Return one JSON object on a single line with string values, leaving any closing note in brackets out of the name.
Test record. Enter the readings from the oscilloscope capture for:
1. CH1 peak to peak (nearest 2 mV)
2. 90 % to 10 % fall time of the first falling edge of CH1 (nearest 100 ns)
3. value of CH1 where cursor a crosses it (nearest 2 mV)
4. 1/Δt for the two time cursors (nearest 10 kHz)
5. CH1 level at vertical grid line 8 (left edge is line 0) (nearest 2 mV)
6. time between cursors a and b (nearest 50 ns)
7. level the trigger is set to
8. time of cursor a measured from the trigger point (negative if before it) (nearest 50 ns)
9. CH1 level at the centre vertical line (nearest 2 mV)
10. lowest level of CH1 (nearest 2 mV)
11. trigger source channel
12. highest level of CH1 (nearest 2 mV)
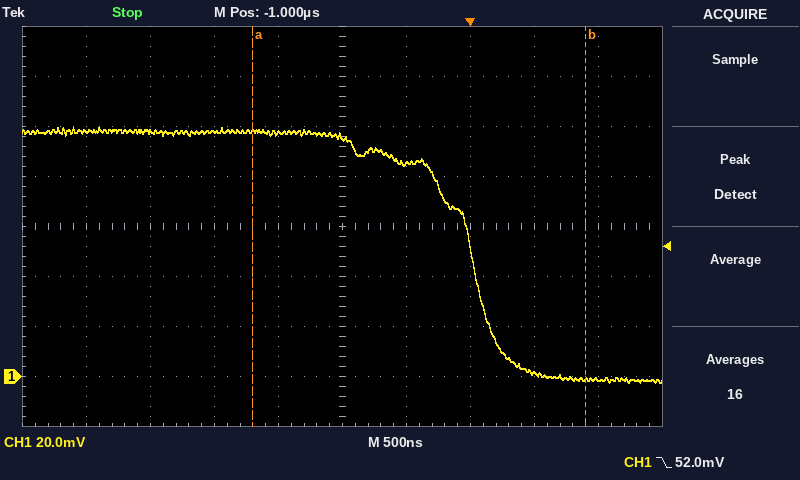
{"CH1 peak to peak": "102 mV", "90 % to 10 % fall time of the first falling edge of CH1": "900 ns", "value of CH1 where cursor a crosses it": "98 mV", "1/Δt for the two time cursors": "380 kHz", "CH1 level at vertical grid line 8 (left edge is line 0)": "2 mV", "time between cursors a and b": "2.60 µs", "level the trigger is set to": "52.0 mV", "time of cursor a measured from the trigger point (negative if before it)": "-1.70 µs", "CH1 level at the centre vertical line": "96 mV", "lowest level of CH1": "-2 mV", "trigger source channel": "CH1", "highest level of CH1": "100 mV"}
